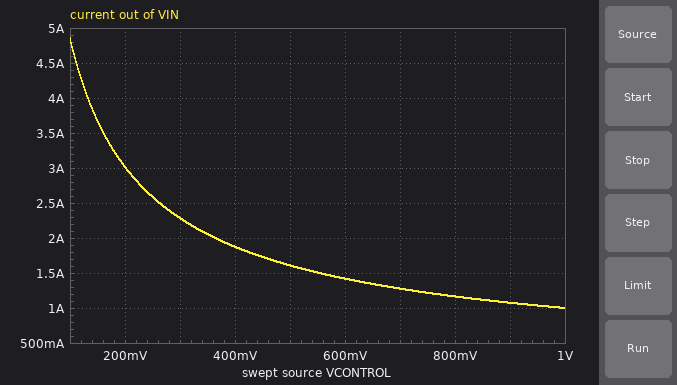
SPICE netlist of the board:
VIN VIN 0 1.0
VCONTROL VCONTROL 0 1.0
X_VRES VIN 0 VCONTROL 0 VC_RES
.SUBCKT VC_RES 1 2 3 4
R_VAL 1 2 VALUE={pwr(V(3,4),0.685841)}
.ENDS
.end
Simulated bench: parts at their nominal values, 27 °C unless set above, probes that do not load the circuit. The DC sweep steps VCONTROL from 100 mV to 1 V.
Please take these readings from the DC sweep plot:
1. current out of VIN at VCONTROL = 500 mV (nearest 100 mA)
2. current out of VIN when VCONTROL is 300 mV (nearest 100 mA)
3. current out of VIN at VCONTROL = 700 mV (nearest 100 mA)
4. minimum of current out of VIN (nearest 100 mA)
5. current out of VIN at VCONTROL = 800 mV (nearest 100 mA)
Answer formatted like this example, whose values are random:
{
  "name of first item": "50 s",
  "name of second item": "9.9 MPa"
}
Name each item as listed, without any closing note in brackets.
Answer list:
{
  "current out of VIN at VCONTROL = 500 mV": "1.6 A",
  "current out of VIN when VCONTROL is 300 mV": "2.3 A",
  "current out of VIN at VCONTROL = 700 mV": "1.3 A",
  "minimum of current out of VIN": "1.0 A",
  "current out of VIN at VCONTROL = 800 mV": "1.2 A"
}
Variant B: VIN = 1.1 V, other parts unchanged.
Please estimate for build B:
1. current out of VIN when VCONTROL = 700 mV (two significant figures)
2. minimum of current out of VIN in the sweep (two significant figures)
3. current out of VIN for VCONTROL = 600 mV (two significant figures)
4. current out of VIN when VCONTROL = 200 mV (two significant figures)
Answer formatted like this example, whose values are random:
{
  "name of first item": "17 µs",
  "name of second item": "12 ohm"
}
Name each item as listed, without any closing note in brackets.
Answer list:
{
  "current out of VIN when VCONTROL = 700 mV": "1.4 A",
  "minimum of current out of VIN in the sweep": "1.1 A",
  "current out of VIN for VCONTROL = 600 mV": "1.6 A",
  "current out of VIN when VCONTROL = 200 mV": "3.3 A"
}
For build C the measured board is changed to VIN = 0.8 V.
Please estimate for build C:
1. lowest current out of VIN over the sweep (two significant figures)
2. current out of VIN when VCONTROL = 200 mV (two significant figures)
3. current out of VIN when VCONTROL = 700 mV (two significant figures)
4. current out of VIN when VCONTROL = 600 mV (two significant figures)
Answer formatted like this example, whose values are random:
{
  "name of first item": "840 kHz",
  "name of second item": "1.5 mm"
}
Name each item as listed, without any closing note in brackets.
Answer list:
{
  "lowest current out of VIN over the sweep": "800 mA",
  "current out of VIN when VCONTROL = 200 mV": "2.4 A",
  "current out of VIN when VCONTROL = 700 mV": "1.0 A",
  "current out of VIN when VCONTROL = 600 mV": "1.1 A"
}
